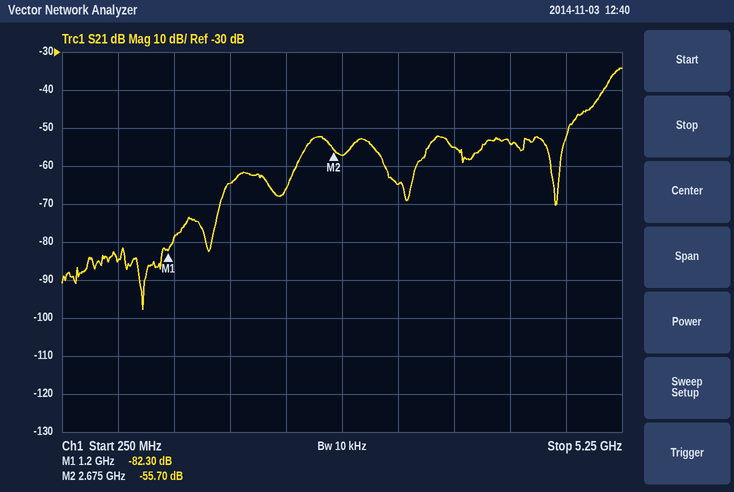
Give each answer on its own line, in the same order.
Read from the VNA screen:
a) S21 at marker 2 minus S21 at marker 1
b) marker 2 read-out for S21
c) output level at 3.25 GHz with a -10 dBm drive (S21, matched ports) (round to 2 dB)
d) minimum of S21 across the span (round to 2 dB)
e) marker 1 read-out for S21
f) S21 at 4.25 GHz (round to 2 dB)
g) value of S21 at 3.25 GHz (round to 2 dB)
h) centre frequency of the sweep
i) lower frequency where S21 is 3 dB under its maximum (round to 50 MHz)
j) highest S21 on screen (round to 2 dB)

26.60 dB
-55.70 dB
-74 dBm
-98 dB
-82.30 dB
-54 dB
-64 dB
2.75 GHz
5.15 GHz
-34 dB
